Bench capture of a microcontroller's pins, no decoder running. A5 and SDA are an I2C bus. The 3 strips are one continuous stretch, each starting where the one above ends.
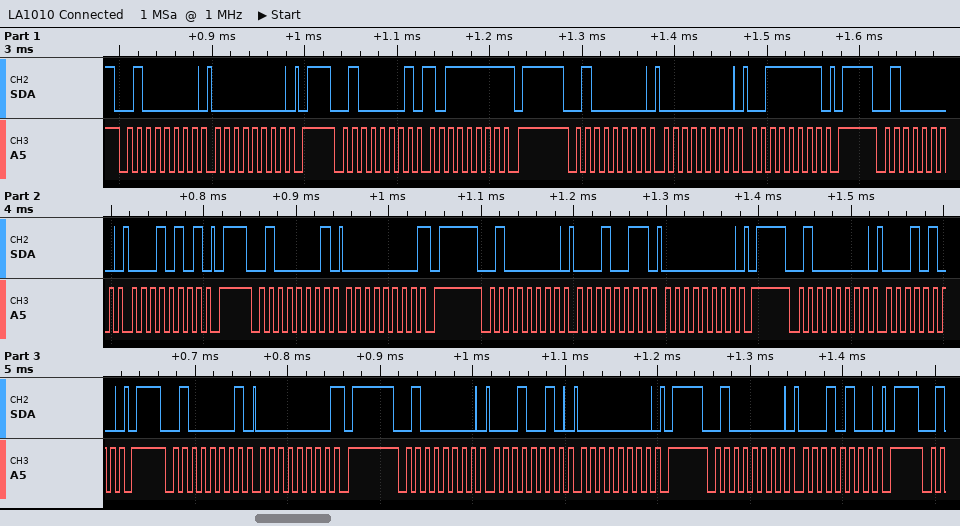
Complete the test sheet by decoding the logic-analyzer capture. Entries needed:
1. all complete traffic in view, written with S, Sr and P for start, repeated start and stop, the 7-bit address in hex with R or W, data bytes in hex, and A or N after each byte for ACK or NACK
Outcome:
S 20W A 00 A P S 20R A BF N P S 20W A 00 A 3F A P S 20W A 15 A P S 20R A 00 N P S 20W A 13 A 00 A P S 20W A 14 A P S 20R A 00 N P S 20W A 12 A 00 A P S 20W A 14 A P
